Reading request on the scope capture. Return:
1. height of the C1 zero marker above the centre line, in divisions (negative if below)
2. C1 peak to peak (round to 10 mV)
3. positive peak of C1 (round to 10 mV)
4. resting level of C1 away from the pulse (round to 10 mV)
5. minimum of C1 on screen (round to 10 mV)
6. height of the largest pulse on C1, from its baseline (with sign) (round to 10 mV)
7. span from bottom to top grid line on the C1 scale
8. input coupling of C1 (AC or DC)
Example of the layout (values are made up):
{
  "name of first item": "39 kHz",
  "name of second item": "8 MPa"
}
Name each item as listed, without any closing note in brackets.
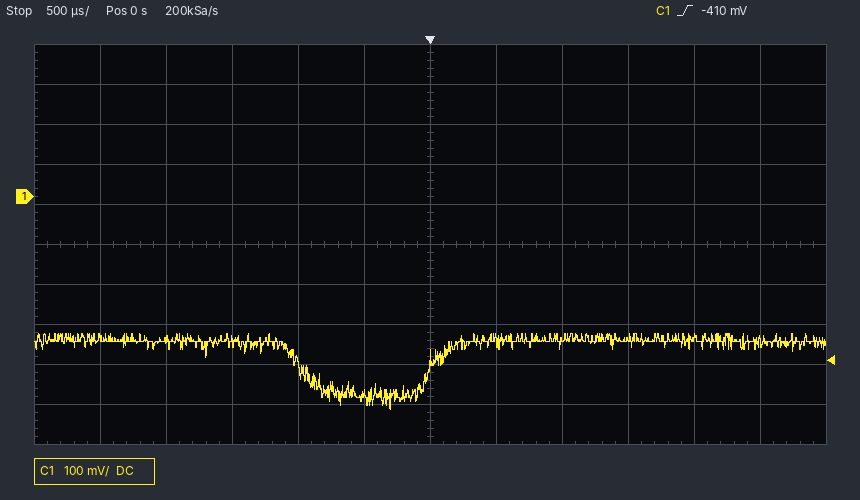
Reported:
{
  "height of the C1 zero marker above the centre line, in divisions": "+1.2 div",
  "C1 peak to peak": "190 mV",
  "positive peak of C1": "-340 mV",
  "resting level of C1 away from the pulse": "-360 mV",
  "minimum of C1 on screen": "-530 mV",
  "height of the largest pulse on C1, from its baseline (with sign)": "-170 mV",
  "span from bottom to top grid line on the C1 scale": "1 V",
  "input coupling of C1": "DC"
}
